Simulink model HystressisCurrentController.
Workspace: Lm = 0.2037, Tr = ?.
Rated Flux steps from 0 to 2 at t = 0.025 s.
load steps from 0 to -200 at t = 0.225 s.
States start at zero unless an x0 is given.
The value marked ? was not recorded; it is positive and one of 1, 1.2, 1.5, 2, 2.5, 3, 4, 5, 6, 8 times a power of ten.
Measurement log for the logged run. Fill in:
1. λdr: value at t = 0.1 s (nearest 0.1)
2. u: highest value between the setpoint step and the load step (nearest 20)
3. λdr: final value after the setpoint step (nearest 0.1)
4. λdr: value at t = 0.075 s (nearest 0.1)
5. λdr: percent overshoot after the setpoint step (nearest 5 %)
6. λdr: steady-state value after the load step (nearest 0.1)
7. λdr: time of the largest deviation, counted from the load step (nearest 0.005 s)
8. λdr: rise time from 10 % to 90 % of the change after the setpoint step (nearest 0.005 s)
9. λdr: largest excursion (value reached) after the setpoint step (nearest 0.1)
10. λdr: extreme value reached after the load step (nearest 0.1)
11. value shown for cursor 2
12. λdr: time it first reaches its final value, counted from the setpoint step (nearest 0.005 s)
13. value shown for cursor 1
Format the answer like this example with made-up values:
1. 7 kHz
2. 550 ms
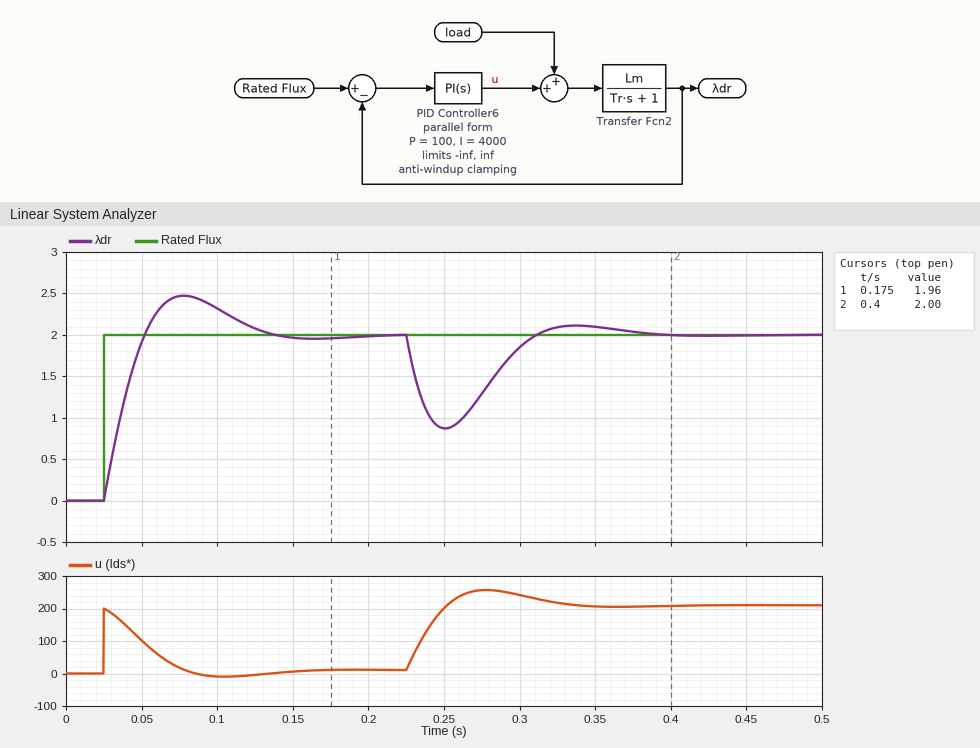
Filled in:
1. 2.3
2. 200
3. 2.0
4. 2.5
5. 25 %
6. 2.0
7. 0.025 s
8. 0.020 s
9. 2.5
10. 0.9
11. 2.00
12. 0.025 s
13. 1.96
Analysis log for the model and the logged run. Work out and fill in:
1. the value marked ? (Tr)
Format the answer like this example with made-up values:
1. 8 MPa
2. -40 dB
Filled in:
1. 0.4
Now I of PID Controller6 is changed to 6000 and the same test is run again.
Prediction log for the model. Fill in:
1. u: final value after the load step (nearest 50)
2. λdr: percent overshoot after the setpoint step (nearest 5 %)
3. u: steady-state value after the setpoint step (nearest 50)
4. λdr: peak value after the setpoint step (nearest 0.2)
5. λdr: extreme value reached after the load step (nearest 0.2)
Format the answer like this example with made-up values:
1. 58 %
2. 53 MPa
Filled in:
1. 200
2. 30 %
3. 0
4. 2.6
5. 1.0
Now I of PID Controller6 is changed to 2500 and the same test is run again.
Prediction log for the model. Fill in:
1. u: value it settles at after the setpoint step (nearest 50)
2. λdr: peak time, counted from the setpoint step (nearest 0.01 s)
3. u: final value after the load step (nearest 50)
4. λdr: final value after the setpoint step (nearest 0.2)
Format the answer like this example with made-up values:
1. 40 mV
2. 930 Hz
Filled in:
1. 0
2. 0.06 s
3. 200
4. 2.0
